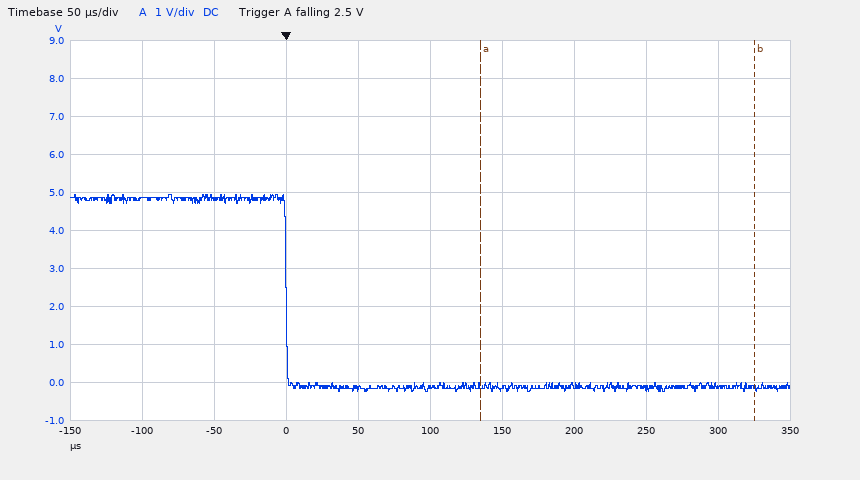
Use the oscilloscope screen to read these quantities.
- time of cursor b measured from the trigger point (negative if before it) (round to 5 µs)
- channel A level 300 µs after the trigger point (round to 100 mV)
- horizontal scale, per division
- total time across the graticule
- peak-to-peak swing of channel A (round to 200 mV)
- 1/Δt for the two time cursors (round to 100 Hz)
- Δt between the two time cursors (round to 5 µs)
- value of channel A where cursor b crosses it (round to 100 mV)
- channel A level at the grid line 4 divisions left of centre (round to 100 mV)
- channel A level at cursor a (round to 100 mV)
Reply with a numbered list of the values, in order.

1. +325 µs
2. -100 mV
3. 50 µs
4. 500 µs
5. 5.2 V
6. 5.3 kHz
7. 190 µs
8. -200 mV
9. 4.8 V
10. -100 mV
